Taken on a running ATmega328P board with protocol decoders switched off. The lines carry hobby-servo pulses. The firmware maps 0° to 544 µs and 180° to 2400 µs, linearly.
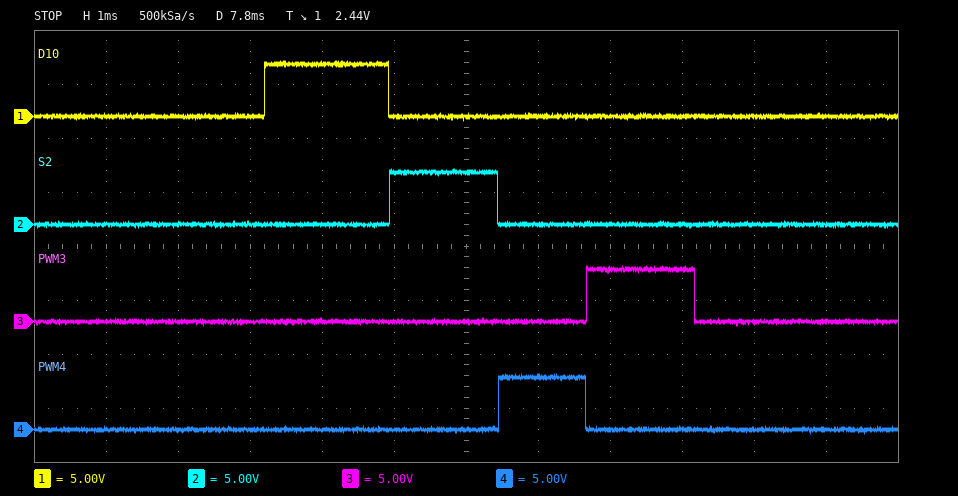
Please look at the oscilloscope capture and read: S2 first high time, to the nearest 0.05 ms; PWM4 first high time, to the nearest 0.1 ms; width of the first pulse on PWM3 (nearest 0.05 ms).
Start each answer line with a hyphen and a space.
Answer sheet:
- 1.50 ms
- 1.2 ms
- 1.50 ms
